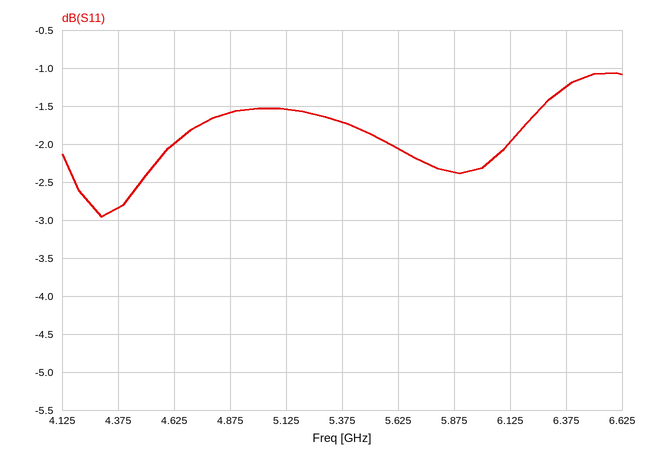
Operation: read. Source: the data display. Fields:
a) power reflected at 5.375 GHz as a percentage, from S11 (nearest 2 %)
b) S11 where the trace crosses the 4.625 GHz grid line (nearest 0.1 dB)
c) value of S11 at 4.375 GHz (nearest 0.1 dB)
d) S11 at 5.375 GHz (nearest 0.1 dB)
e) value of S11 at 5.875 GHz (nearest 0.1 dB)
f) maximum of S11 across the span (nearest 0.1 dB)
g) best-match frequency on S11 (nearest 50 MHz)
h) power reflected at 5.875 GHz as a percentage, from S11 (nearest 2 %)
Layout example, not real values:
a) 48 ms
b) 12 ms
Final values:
a) 68 %
b) -2.0 dB
c) -2.8 dB
d) -1.7 dB
e) -2.4 dB
f) -1.1 dB
g) 4.30 GHz
h) 58 %
